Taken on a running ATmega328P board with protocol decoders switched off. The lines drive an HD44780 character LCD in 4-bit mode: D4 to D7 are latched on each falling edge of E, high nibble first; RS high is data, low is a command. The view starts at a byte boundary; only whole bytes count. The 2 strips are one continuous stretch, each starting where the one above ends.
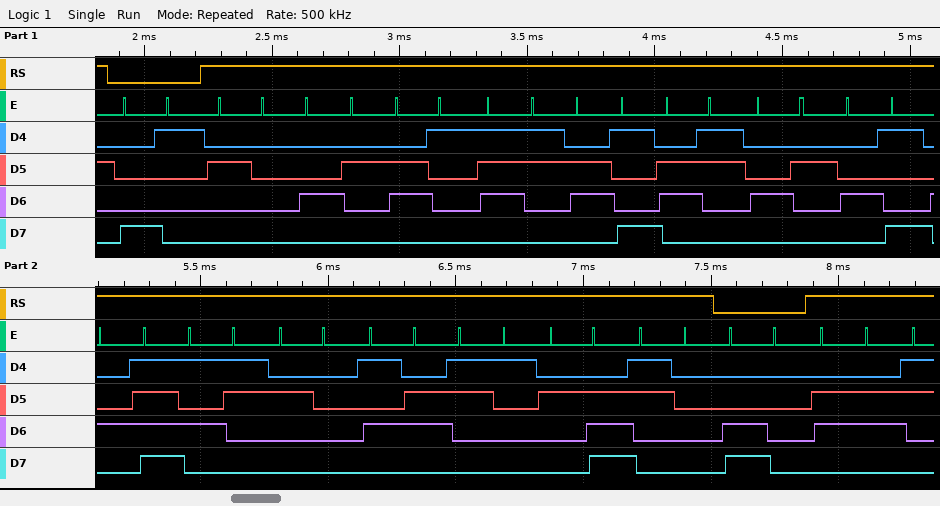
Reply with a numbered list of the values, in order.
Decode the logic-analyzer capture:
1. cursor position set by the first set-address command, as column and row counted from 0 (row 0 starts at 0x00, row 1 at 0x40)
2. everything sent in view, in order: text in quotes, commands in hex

1. column 1, row 0
2. 0x81 " BasicBIOS V1.0" 0xC0 "f"
